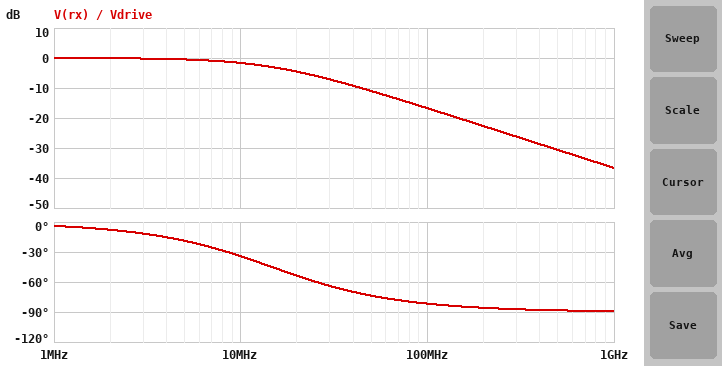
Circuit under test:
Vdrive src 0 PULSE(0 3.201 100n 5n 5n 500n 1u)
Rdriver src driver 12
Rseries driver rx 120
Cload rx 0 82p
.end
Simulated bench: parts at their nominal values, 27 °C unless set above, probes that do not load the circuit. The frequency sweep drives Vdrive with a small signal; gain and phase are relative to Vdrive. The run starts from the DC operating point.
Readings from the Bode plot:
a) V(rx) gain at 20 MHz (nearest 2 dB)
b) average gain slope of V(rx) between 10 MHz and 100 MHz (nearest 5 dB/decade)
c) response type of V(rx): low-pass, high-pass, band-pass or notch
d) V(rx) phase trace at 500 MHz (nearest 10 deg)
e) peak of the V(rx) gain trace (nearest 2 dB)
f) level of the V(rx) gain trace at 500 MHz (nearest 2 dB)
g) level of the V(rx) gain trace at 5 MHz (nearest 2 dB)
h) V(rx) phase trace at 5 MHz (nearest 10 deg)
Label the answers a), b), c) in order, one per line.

a) -4 dB
b) -15 dB/decade
c) low-pass
d) -90 deg
e) 0 dB
f) -30 dB
g) 0 dB
h) -20 deg
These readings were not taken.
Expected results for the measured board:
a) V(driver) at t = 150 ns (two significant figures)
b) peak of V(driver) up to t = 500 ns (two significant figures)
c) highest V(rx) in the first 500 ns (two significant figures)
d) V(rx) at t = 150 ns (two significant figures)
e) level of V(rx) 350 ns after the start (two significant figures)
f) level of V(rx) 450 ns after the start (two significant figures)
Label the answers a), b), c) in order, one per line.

a) 3.2 V
b) 3.2 V
c) 3.2 V
d) 3.2 V
e) 3.2 V
f) 3.2 V
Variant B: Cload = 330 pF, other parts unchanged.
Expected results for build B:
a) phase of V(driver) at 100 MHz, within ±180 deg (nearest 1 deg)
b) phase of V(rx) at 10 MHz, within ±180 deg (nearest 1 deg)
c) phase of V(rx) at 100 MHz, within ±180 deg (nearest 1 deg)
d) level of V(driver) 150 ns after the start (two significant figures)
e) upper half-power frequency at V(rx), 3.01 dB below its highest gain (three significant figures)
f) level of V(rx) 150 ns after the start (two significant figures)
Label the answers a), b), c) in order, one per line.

a) 0 deg
b) -70 deg
c) -88 deg
d) 3.1 V
e) 3.65 MHz
f) 2.1 V
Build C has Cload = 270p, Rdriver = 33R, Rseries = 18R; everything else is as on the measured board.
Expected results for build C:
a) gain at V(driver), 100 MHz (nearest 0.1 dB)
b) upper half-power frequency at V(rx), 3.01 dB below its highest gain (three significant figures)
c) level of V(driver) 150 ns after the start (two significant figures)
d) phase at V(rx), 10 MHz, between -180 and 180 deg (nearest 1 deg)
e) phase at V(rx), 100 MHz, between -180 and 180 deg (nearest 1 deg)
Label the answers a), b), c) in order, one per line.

a) -8.7 dB
b) 11.6 MHz
c) 3.1 V
d) -41 deg
e) -83 deg
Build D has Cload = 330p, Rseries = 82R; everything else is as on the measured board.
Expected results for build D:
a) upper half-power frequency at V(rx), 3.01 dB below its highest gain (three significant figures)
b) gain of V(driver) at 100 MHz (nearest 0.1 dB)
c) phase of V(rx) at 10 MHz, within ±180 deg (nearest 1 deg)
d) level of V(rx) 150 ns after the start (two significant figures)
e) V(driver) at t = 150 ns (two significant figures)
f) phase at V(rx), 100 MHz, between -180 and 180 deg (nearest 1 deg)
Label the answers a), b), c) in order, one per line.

a) 5.13 MHz
b) -1.2 dB
c) -63 deg
d) 2.5 V
e) 3.1 V
f) -87 deg
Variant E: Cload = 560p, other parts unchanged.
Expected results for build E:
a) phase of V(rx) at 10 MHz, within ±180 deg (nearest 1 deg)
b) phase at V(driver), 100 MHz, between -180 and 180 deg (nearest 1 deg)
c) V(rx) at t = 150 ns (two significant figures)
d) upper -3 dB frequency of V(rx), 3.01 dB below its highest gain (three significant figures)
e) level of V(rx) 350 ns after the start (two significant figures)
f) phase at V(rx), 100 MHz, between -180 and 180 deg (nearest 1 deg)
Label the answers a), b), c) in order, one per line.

a) -78 deg
b) 0 deg
c) 1.5 V
d) 2.15 MHz
e) 3.1 V
f) -89 deg
